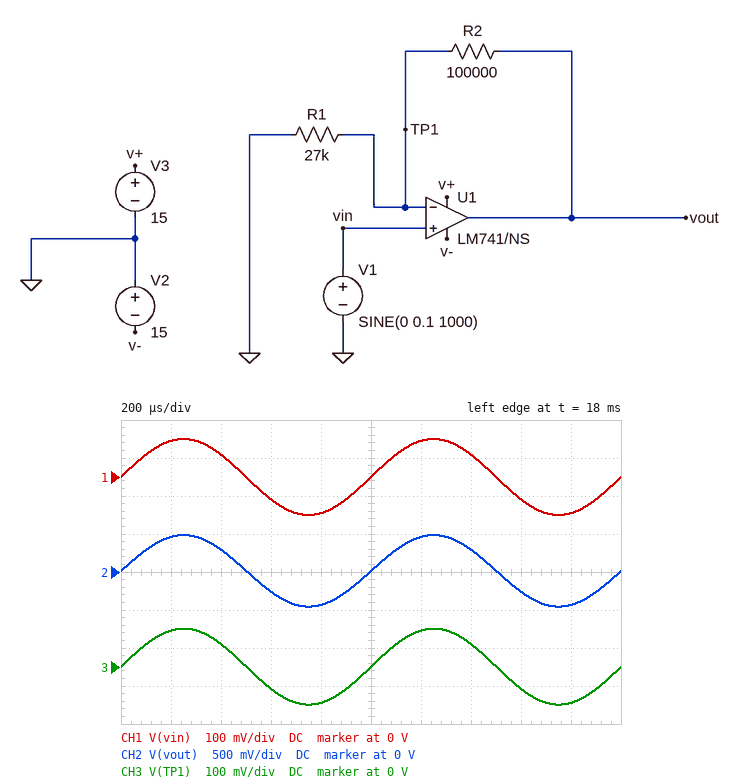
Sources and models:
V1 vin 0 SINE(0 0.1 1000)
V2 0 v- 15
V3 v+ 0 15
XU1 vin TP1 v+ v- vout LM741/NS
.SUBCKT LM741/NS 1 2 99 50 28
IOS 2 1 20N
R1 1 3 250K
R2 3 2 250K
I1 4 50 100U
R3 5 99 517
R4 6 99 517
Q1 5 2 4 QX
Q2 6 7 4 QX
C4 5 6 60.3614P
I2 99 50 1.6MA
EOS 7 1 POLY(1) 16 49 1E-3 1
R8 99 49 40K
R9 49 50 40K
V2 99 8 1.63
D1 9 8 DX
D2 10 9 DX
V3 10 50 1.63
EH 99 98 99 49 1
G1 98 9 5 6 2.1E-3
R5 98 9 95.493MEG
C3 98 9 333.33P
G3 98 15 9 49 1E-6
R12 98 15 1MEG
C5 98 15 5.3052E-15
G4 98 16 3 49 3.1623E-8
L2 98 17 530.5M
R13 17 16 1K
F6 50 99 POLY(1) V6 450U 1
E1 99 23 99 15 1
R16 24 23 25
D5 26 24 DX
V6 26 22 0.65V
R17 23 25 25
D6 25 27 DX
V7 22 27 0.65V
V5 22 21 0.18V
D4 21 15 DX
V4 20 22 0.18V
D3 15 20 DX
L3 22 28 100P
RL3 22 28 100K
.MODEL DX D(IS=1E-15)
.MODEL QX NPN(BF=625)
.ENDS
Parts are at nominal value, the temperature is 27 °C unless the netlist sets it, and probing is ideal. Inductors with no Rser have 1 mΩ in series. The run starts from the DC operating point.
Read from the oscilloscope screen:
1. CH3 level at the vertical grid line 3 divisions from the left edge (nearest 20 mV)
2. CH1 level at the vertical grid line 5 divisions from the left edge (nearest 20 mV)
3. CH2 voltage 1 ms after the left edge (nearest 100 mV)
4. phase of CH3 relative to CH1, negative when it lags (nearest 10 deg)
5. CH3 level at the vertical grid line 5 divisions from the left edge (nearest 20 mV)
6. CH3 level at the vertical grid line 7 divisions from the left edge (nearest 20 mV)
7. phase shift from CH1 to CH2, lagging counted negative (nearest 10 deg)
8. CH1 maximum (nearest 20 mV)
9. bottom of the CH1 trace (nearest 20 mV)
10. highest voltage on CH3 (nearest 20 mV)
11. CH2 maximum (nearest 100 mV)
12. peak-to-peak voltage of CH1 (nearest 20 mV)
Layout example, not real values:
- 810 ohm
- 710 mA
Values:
- -60 mV
- 0 V
- 0 V
- 0 deg
- 0 V
- 60 mV
- 0 deg
- 100 mV
- -100 mV
- 100 mV
- 500 mV
- 200 mV
